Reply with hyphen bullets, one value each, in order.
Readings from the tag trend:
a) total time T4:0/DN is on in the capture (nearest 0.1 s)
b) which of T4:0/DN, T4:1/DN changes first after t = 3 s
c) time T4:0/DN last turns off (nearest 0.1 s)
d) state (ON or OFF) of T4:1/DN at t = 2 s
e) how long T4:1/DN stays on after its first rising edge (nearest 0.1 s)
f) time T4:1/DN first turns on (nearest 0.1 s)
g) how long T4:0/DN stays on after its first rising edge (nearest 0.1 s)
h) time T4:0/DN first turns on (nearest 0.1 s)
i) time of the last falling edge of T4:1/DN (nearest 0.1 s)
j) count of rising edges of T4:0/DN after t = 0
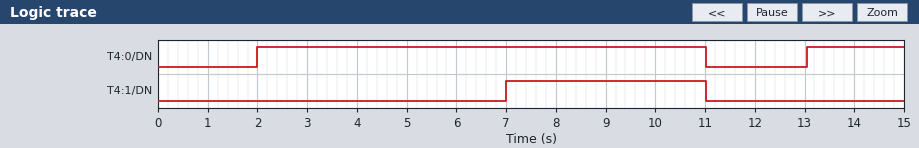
- 11.0 s
- T4:1/DN
- 11.0 s
- OFF
- 4.0 s
- 7.0 s
- 9.0 s
- 2.0 s
- 11.0 s
- 2
